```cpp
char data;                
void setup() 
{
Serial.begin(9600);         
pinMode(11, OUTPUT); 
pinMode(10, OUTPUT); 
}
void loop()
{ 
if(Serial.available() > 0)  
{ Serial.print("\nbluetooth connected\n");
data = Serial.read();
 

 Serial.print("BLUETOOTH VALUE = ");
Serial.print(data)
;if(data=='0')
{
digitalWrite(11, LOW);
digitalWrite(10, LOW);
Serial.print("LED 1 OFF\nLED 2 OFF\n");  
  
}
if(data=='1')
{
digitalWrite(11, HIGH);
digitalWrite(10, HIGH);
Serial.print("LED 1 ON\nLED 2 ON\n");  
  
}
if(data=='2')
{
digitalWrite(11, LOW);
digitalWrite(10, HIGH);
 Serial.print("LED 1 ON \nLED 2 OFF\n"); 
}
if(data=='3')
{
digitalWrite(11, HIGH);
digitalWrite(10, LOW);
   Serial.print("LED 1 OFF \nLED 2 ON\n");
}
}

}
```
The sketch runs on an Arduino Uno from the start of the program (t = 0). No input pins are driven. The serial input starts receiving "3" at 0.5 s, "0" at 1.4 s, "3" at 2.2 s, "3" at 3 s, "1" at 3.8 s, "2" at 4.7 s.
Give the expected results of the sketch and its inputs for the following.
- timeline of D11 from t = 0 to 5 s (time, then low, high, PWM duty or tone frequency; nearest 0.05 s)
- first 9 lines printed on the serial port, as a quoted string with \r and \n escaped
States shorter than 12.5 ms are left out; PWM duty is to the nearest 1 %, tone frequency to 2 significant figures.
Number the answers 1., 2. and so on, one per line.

1. 0 s low; 0.5 s high; 1.4 s low; 2.2 s high; 4.7 s low
2. "\nbluetooth connected\nBLUETOOTH VALUE = 3LED 1 OFF \nLED 2 ON\n\nbluetooth connected\nBLUETOOTH VALUE = 0LED 1 OFF\nLED 2 OFF\n\n"
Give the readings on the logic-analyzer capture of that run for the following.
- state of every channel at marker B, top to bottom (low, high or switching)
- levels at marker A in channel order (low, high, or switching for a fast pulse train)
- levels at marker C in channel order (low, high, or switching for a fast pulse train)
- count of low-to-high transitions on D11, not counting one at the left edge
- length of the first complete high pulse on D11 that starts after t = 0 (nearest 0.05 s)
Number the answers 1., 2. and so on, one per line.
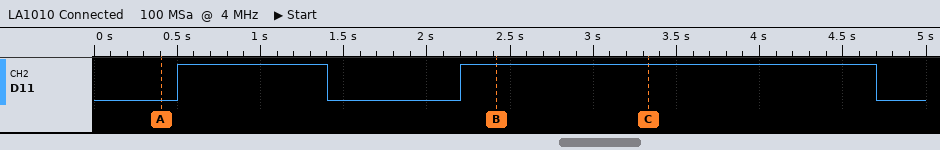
1. D11 high
2. D11 low
3. D11 high
4. 2
5. 0.90 s
